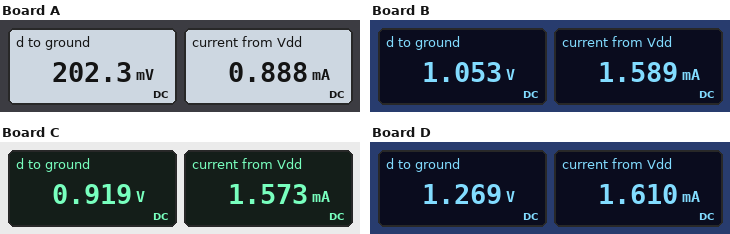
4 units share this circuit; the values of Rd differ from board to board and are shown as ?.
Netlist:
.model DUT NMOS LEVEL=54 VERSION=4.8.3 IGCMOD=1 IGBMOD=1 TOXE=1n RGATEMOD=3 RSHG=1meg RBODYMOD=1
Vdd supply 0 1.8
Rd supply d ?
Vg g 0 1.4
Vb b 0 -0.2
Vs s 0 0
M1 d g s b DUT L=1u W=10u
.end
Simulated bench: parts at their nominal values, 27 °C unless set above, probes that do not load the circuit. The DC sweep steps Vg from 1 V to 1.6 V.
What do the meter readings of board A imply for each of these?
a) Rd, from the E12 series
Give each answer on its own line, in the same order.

1.8 kΩ
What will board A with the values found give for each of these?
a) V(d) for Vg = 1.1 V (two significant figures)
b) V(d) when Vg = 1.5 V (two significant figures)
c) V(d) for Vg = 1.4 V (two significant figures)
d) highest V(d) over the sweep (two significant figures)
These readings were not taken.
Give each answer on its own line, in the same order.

220 mV
200 mV
200 mV
230 mV
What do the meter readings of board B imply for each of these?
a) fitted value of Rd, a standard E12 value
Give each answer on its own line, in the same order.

470 Ω
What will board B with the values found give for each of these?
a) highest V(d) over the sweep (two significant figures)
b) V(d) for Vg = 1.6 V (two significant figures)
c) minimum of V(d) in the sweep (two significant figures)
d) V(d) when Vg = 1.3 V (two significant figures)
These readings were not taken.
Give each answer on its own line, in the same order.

1.2 V
1.0 V
1.0 V
1.1 V
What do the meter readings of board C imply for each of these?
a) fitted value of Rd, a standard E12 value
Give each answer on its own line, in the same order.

560 Ω
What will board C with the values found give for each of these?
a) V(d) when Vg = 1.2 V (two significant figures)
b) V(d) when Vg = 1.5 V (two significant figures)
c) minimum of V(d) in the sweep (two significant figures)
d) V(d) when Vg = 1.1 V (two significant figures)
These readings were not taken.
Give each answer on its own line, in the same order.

980 mV
890 mV
870 mV
1.0 V
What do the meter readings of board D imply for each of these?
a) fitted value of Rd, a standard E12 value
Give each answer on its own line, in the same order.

330 Ω
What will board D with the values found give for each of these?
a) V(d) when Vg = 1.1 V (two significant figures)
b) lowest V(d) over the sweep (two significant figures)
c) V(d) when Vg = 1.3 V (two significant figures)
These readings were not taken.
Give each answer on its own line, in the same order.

1.3 V
1.2 V
1.3 V
